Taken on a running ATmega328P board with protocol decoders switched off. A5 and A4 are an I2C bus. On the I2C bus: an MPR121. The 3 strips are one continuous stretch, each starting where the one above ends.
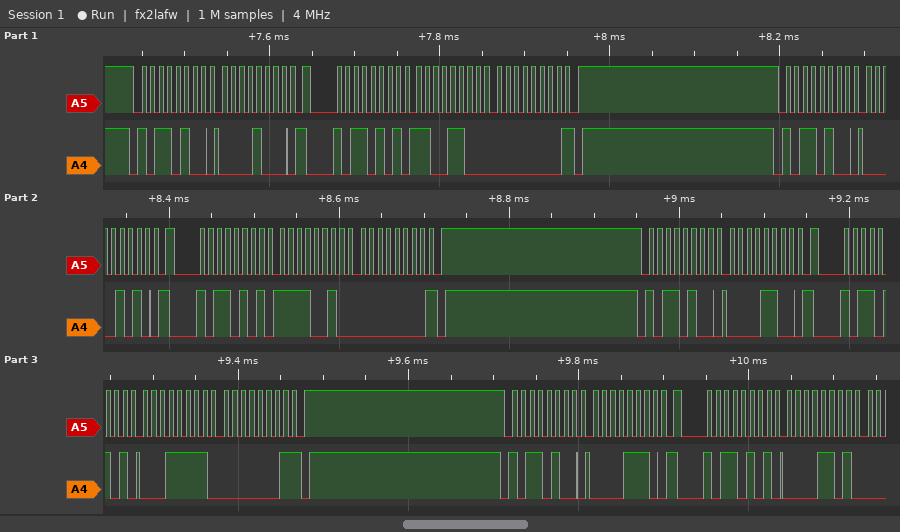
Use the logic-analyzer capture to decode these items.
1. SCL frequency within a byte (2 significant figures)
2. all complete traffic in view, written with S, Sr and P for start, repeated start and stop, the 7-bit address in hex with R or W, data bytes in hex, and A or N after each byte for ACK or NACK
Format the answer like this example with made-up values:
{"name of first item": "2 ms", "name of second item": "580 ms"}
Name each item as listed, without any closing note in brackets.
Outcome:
{"SCL frequency within a byte": "100 kHz", "all complete traffic in view, written with S, Sr and P for start, repeated start and stop, the 7-bit address in hex with R or W, data bytes in hex, and A or N after each byte for ACK or NACK": "S 5AW A 08 A Sr 5AR A CC A 00 N P S 5AW A 0A A Sr 5AR A F2 A 00 N P S 5AW A 0C A Sr 5AR A 1F A 01 N P S 5AW A 0E A Sr 5AR A 0D A"}
